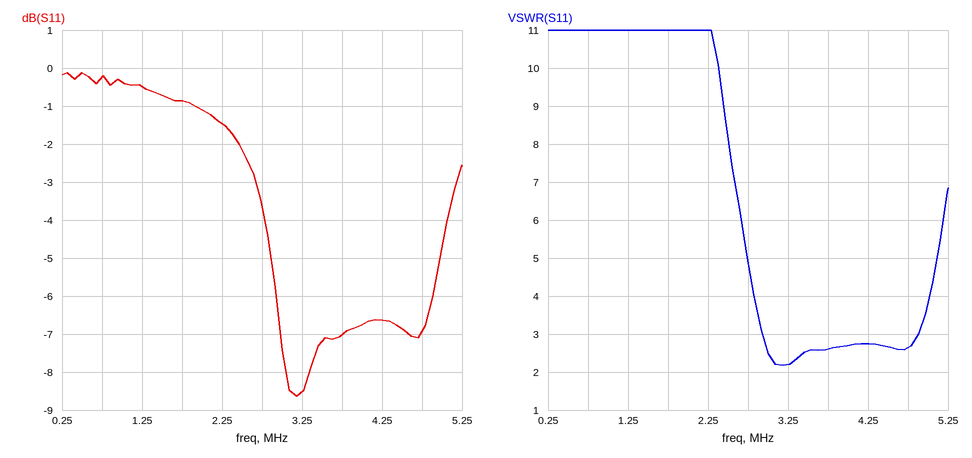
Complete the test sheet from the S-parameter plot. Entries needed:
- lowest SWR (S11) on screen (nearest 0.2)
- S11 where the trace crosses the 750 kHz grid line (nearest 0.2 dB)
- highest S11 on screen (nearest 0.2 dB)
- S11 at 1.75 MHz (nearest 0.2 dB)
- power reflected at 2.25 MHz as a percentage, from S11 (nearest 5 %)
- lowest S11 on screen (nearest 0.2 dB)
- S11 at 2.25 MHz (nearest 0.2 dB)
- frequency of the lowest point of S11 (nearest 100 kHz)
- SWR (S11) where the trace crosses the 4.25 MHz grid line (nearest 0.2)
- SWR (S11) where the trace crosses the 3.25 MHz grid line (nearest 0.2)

2.2
-0.2 dB
-0.2 dB
-0.8 dB
70 %
-8.6 dB
-1.4 dB
3.2 MHz
2.8
2.2
